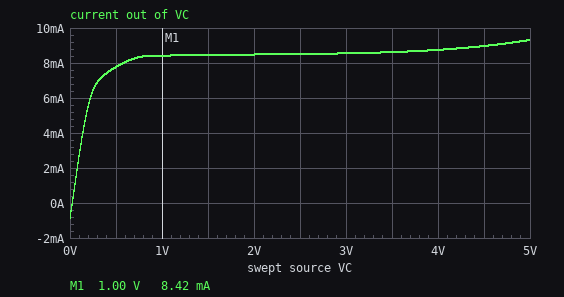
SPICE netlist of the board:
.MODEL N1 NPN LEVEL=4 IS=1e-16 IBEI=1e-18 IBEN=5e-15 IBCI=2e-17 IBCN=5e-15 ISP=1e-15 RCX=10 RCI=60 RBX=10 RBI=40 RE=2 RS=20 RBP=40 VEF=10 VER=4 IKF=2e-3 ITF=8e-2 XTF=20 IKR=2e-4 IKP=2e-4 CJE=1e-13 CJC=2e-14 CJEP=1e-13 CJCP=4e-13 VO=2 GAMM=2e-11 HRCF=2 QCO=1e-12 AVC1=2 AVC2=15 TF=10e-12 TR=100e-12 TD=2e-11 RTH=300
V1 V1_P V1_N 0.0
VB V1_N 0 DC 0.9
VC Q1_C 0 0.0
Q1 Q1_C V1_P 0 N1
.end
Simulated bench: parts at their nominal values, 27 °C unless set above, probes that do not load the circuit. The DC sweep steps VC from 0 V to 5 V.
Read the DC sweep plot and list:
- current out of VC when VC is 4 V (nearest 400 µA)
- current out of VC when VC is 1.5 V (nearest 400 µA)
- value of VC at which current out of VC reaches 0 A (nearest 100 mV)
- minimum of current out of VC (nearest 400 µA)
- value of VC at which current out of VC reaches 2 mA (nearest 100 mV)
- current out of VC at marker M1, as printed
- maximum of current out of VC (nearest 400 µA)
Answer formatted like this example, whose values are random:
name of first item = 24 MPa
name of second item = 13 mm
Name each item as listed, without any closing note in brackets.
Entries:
current out of VC when VC is 4 V = 8.8 mA
current out of VC when VC is 1.5 V = 8.4 mA
value of VC at which current out of VC reaches 0 A = 0 V
minimum of current out of VC = -800 µA
value of VC at which current out of VC reaches 2 mA = 100 mV
current out of VC at marker M1, as printed = 8.42 mA
maximum of current out of VC = 9.2 mA
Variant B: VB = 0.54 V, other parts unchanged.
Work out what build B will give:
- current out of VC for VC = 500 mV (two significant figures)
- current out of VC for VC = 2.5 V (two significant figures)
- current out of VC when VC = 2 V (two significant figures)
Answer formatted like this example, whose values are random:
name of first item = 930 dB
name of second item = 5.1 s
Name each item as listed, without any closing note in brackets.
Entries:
current out of VC for VC = 500 mV = 100 nA
current out of VC for VC = 2.5 V = 120 nA
current out of VC when VC = 2 V = 110 nA
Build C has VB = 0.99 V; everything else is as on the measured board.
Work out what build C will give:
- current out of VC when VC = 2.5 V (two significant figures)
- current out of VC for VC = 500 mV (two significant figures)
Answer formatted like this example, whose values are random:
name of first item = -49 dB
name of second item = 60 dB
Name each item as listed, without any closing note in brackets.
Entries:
current out of VC when VC = 2.5 V = 20 mA
current out of VC for VC = 500 mV = 15 mA
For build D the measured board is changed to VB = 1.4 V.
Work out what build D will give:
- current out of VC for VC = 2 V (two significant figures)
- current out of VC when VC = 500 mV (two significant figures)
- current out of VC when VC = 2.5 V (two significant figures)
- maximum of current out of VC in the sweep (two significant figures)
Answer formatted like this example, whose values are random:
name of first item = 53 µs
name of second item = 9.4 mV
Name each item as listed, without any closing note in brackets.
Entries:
current out of VC for VC = 2 V = 34 mA
current out of VC when VC = 500 mV = 25 mA
current out of VC when VC = 2.5 V = 36 mA
maximum of current out of VC in the sweep = 46 mA
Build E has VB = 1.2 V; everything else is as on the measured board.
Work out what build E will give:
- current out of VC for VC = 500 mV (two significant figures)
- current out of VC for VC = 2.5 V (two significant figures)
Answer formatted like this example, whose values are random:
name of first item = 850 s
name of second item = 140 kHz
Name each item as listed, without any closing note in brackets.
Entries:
current out of VC for VC = 500 mV = 23 mA
current out of VC for VC = 2.5 V = 34 mA
